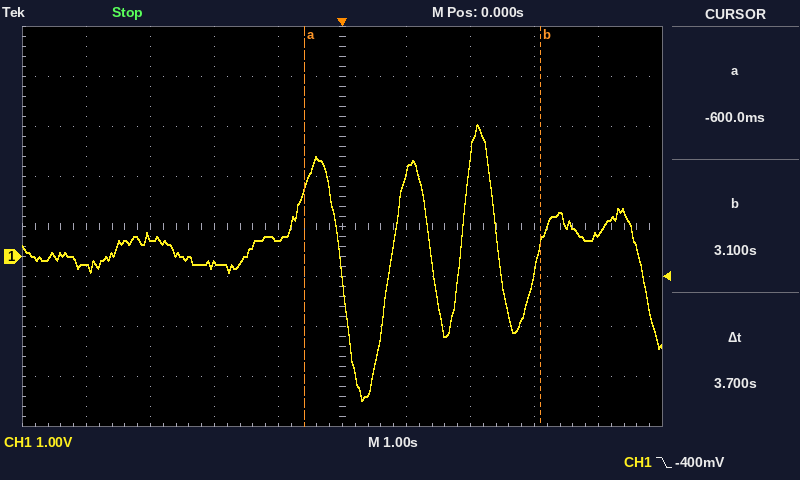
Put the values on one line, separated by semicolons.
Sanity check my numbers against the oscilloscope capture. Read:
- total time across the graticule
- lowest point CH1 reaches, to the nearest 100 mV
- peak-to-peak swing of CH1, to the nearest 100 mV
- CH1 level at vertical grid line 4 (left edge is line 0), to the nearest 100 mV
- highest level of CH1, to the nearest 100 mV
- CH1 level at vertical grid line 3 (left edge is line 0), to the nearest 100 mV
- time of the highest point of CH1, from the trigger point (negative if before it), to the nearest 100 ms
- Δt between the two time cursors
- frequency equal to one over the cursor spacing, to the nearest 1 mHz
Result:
10 s; -2.9 V; 5.5 V; 300 mV; 2.6 V; -200 mV; +2.1 s; 3.7 s; 270 mHz
